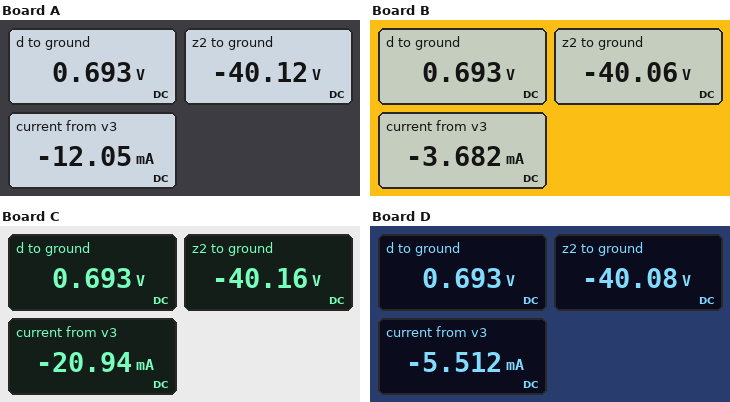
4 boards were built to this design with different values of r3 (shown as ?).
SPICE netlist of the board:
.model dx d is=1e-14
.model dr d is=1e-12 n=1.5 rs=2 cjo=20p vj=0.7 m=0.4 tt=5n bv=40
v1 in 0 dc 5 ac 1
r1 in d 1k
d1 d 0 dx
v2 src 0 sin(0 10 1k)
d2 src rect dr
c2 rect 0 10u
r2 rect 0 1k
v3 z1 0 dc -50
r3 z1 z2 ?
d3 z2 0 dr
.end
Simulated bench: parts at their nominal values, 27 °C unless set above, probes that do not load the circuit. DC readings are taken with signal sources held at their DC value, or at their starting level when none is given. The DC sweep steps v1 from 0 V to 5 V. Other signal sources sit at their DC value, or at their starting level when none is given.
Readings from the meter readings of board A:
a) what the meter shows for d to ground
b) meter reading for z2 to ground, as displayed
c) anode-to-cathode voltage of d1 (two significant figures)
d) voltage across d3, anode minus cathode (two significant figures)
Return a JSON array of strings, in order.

["0.693 V", "-40.12 V", "690 mV", "-40 V"]
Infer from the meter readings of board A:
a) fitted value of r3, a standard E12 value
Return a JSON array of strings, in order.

["820 Ω"]
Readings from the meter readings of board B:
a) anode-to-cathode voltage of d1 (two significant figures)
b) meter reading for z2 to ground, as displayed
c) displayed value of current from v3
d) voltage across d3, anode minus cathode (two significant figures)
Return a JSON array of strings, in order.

["690 mV", "-40.06 V", "-3.682 mA", "-40 V"]
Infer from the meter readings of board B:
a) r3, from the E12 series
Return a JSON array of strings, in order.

["2.7 kΩ"]
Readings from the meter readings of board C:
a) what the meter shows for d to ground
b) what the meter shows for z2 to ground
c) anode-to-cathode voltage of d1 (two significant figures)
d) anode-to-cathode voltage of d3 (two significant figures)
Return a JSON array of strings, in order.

["0.693 V", "-40.16 V", "690 mV", "-40 V"]
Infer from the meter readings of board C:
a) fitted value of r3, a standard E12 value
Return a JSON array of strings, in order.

["470 Ω"]
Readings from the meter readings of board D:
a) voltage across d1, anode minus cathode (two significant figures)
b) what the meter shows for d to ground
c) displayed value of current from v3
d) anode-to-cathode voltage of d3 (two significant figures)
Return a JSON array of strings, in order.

["690 mV", "0.693 V", "-5.512 mA", "-40 V"]
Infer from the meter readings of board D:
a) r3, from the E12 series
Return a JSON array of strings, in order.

["1.8 kΩ"]
